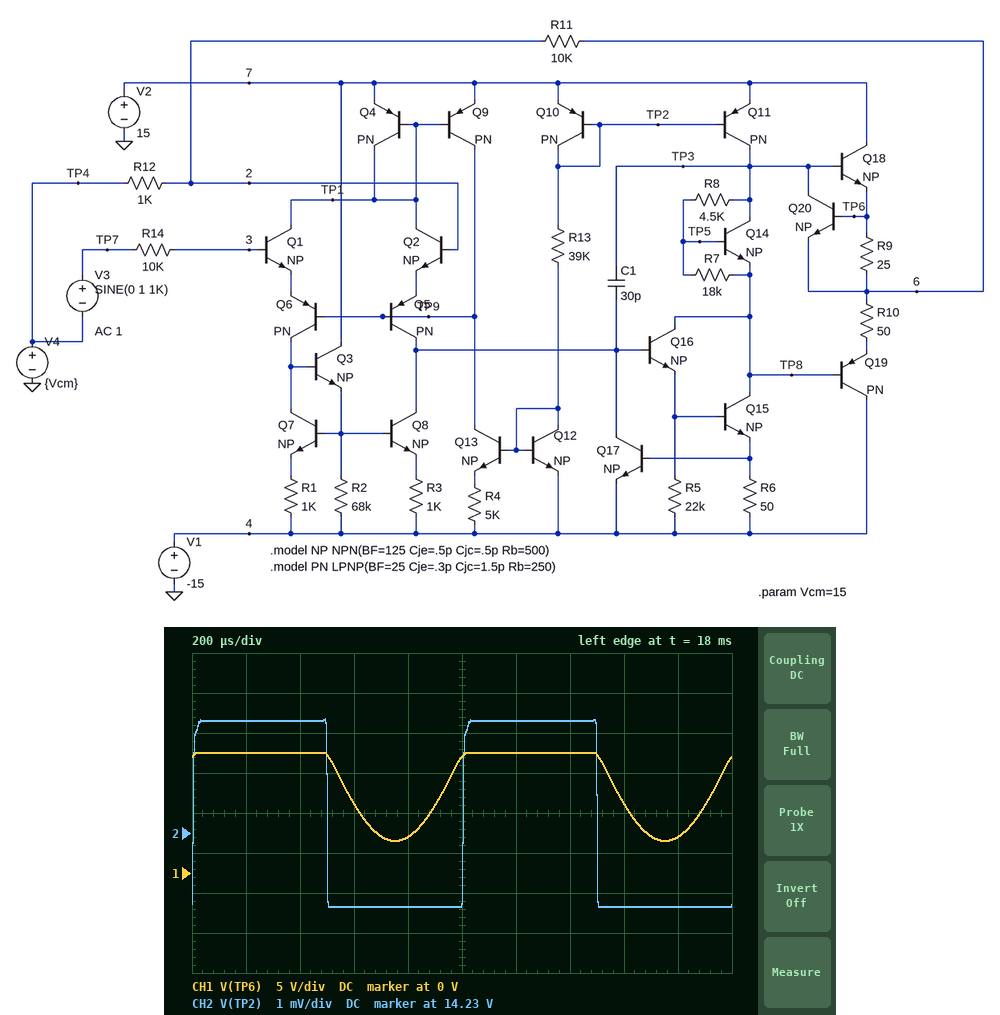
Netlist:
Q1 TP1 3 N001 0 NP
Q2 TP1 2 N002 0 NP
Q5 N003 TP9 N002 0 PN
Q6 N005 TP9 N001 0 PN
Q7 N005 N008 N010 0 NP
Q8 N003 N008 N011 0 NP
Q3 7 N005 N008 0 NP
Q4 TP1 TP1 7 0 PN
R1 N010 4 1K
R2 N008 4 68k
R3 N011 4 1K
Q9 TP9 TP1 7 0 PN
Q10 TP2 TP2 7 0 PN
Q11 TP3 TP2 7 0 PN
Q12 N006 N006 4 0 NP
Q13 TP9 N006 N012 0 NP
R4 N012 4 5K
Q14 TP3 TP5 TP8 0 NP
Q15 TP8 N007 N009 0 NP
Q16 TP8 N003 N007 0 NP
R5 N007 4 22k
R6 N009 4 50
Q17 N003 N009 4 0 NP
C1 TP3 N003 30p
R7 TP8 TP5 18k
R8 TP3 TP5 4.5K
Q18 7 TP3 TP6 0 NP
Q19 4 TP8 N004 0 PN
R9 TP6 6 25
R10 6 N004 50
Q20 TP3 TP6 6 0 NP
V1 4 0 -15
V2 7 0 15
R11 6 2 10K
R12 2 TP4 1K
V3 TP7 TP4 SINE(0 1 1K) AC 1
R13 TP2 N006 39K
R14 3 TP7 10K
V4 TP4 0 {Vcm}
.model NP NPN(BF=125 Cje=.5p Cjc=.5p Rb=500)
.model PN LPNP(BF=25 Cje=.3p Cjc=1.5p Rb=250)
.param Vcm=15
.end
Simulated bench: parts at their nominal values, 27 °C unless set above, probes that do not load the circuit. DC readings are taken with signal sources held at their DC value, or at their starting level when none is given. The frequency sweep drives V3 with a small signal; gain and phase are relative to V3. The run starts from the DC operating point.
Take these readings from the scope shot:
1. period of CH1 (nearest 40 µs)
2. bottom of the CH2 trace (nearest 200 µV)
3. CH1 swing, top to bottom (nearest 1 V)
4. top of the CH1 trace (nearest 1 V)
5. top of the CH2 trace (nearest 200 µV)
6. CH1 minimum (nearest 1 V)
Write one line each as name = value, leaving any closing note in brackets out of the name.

period of CH1 = 1.00 ms
bottom of the CH2 trace = 14.2292 V
CH1 swing, top to bottom = 11 V
top of the CH1 trace = 15 V
top of the CH2 trace = 14.2338 V
CH1 minimum = 4 V
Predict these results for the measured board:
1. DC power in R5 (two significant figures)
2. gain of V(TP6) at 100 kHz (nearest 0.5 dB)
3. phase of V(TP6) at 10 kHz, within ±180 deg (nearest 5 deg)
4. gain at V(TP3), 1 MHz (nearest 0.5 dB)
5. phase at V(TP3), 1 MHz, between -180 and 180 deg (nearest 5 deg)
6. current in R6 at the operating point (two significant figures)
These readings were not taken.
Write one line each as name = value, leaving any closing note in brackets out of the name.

DC power in R5 = 28 µW
gain of V(TP6) at 100 kHz = 10.0 dB
phase of V(TP6) at 10 kHz, within ±180 deg = -5 deg
gain at V(TP3), 1 MHz = -10.0 dB
phase at V(TP3), 1 MHz, between -180 and 180 deg = -90 deg
current in R6 at the operating point = 530 µA
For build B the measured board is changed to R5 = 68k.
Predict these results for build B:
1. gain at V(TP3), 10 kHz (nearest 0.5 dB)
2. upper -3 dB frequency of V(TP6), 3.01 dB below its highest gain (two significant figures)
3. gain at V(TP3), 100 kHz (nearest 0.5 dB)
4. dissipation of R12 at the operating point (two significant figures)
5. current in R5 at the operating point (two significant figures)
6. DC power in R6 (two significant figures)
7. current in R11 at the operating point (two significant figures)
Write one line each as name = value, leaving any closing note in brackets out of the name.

gain at V(TP3), 10 kHz = 12.5 dB
upper -3 dB frequency of V(TP6), 3.01 dB below its highest gain = 80 kHz
gain at V(TP3), 100 kHz = 8.5 dB
dissipation of R12 at the operating point = 1.5 µW
current in R5 at the operating point = 12 µA
DC power in R6 = 17 µW
current in R11 at the operating point = 35 µA
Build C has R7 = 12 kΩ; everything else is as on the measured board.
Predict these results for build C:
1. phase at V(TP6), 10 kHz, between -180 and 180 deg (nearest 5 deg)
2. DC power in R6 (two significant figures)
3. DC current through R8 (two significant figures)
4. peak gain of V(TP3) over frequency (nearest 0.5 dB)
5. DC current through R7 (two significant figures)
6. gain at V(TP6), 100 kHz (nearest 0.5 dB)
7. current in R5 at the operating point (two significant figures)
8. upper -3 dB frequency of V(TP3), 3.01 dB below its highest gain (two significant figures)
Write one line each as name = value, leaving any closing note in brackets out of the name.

phase at V(TP6), 10 kHz, between -180 and 180 deg = -5 deg
DC power in R6 = 2.8 µW
DC current through R8 = 63 µA
peak gain of V(TP3) over frequency = 6.0 dB
DC current through R7 = 61 µA
gain at V(TP6), 100 kHz = 11.0 dB
current in R5 at the operating point = 34 µA
upper -3 dB frequency of V(TP3), 3.01 dB below its highest gain = 92 kHz
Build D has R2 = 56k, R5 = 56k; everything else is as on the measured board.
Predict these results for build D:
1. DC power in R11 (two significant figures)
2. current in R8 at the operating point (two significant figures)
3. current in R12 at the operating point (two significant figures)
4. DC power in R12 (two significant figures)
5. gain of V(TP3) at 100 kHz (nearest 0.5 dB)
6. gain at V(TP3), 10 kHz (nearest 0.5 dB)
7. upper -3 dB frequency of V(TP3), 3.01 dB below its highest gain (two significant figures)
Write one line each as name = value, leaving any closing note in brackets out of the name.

DC power in R11 = 12 µW
current in R8 at the operating point = 47 µA
current in R12 at the operating point = 39 µA
DC power in R12 = 1.5 µW
gain of V(TP3) at 100 kHz = 8.5 dB
gain at V(TP3), 10 kHz = 12.5 dB
upper -3 dB frequency of V(TP3), 3.01 dB below its highest gain = 80 kHz
